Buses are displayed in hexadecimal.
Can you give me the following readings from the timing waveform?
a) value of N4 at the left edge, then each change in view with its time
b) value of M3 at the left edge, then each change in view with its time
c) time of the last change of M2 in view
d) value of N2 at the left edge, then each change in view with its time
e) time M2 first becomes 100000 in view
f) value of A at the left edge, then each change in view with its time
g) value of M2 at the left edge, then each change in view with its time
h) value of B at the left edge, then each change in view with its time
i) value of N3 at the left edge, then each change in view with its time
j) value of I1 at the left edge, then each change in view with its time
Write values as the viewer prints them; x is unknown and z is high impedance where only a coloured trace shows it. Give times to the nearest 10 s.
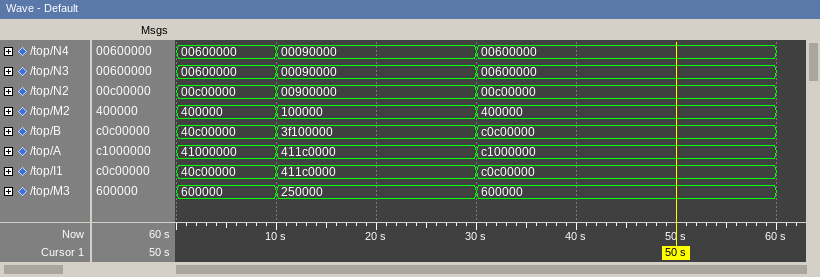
00600000, 00090000 at 10 s, 00600000 at 30 s
600000, 250000 at 10 s, 600000 at 30 s
30 s
00c00000, 00900000 at 10 s, 00c00000 at 30 s
10 s
41000000, 411c0000 at 10 s, c1000000 at 30 s
400000, 100000 at 10 s, 400000 at 30 s
40c00000, 3f100000 at 10 s, c0c00000 at 30 s
00600000, 00090000 at 10 s, 00600000 at 30 s
40c00000, 411c0000 at 10 s, c0c00000 at 30 s
